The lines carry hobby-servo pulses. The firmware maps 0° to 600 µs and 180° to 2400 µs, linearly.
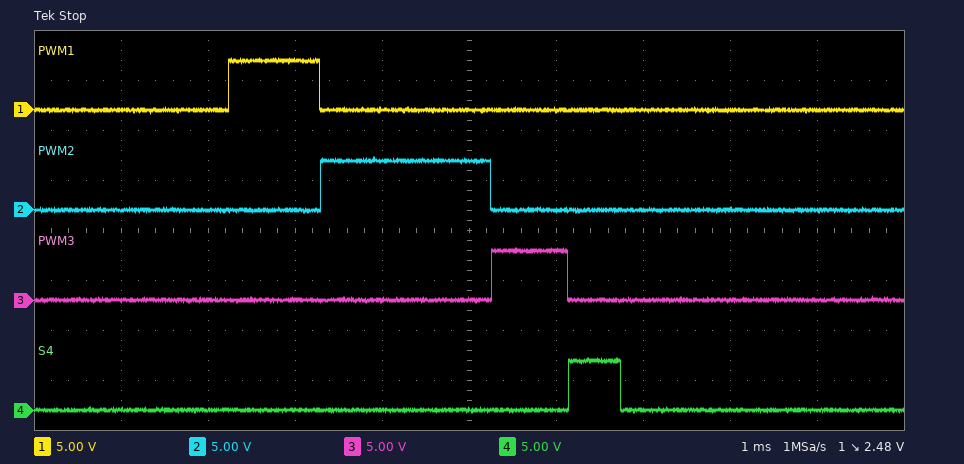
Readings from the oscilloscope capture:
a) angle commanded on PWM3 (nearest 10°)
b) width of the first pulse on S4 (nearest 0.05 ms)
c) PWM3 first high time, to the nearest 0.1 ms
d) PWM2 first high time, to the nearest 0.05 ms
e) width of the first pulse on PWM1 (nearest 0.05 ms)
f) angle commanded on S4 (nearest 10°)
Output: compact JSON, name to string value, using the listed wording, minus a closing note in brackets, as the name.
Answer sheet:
{"angle commanded on PWM3": "30°", "width of the first pulse on S4": "0.60 ms", "PWM3 first high time, to the nearest 0.1 ms": "0.9 ms", "PWM2 first high time, to the nearest 0.05 ms": "1.95 ms", "width of the first pulse on PWM1": "1.05 ms", "angle commanded on S4": "0°"}
